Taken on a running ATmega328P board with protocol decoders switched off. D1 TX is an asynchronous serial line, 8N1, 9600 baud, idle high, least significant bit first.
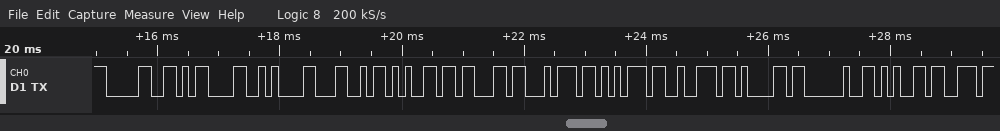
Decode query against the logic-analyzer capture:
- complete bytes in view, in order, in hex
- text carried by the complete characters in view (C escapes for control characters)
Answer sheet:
30 0D 0A 4C 65 63 74 75 72 61 20 65
"0\r\nLectura e"
